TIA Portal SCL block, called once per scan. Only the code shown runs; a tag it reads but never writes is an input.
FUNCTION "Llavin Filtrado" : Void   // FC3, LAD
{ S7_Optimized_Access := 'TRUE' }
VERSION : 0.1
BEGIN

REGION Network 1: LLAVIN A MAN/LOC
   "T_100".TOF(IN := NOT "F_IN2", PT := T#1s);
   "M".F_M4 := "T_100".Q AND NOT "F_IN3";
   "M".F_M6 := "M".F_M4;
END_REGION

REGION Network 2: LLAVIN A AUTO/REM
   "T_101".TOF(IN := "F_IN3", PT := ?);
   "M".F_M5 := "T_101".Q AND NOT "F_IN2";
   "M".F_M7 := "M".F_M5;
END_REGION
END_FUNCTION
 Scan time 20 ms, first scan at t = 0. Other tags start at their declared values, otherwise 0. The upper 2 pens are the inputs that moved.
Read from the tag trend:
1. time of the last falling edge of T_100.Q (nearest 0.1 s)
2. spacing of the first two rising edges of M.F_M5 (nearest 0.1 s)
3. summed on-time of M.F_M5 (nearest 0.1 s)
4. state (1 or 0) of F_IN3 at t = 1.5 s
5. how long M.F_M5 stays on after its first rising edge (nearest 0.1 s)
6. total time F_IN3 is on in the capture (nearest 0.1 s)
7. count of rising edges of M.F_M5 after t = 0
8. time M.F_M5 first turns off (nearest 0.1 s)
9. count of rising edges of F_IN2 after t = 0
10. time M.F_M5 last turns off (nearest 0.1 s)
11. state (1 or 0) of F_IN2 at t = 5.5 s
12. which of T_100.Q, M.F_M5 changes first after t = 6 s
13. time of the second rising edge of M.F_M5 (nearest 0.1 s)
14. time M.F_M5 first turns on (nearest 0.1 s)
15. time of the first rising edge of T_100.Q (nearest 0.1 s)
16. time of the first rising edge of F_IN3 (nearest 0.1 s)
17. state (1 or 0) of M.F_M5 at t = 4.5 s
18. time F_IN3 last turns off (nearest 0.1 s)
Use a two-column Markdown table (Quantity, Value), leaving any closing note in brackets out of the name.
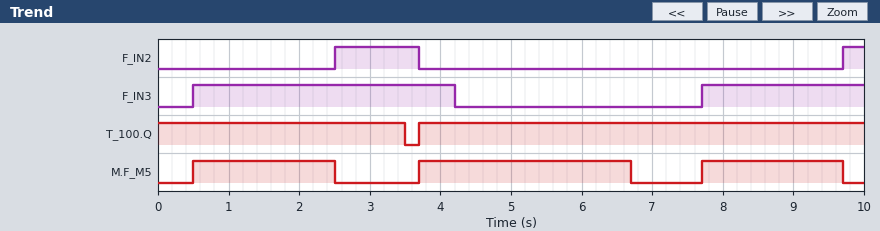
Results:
| Quantity | Value |
|---|---|
| time of the last falling edge of T_100.Q | 3.5 s |
| spacing of the first two rising edges of M.F_M5 | 3.2 s |
| summed on-time of M.F_M5 | 7.0 s |
| state (1 or 0) of F_IN3 at t = 1.5 s | 1 |
| how long M.F_M5 stays on after its first rising edge | 2.0 s |
| total time F_IN3 is on in the capture | 6.0 s |
| count of rising edges of M.F_M5 after t = 0 | 3 |
| time M.F_M5 first turns off | 2.5 s |
| count of rising edges of F_IN2 after t = 0 | 2 |
| time M.F_M5 last turns off | 9.7 s |
| state (1 or 0) of F_IN2 at t = 5.5 s | 0 |
| which of T_100.Q, M.F_M5 changes first after t = 6 s | M.F_M5 |
| time of the second rising edge of M.F_M5 | 3.7 s |
| time M.F_M5 first turns on | 0.5 s |
| time of the first rising edge of T_100.Q | 3.7 s |
| time of the first rising edge of F_IN3 | 0.5 s |
| state (1 or 0) of M.F_M5 at t = 4.5 s | 1 |
| time F_IN3 last turns off | 4.2 s |
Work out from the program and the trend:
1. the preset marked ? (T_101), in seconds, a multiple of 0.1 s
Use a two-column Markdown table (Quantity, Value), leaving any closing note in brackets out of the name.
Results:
| Quantity | Value |
|---|---|
| the preset marked ? (T_101), in seconds, a multiple of 0.1 s | 2.5 s |
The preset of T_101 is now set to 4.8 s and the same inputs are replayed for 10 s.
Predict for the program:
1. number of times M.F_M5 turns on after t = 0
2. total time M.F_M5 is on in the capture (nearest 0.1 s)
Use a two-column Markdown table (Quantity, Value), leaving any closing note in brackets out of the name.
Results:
| Quantity | Value |
|---|---|
| number of times M.F_M5 turns on after t = 0 | 2 |
| total time M.F_M5 is on in the capture | 8.0 s |
